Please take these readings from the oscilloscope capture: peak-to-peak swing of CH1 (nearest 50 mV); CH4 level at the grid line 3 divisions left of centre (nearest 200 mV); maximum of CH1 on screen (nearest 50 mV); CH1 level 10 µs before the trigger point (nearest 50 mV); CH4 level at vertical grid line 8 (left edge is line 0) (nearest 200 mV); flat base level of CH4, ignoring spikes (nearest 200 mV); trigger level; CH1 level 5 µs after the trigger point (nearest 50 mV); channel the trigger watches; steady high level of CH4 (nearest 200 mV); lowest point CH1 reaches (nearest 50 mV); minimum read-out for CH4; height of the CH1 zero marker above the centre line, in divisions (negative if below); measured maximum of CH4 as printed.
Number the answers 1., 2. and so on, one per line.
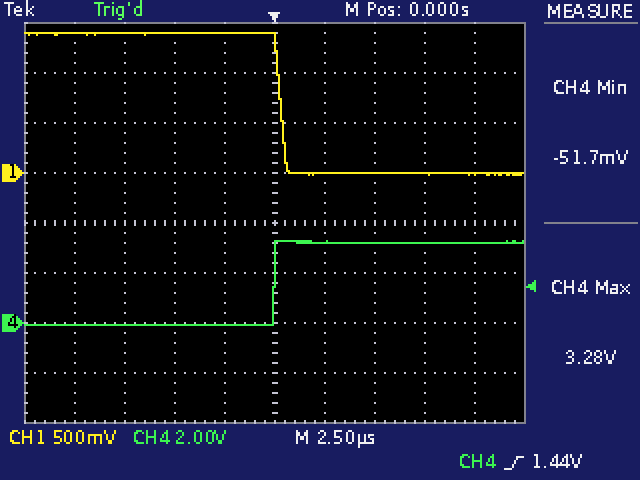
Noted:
1. 1.40 V
2. 0.0 V
3. 1.40 V
4. 1.40 V
5. 3.2 V
6. 0.0 V
7. 1.44 V
8. 0 mV
9. CH4
10. 3.2 V
11. 0 mV
12. -51.7 mV
13. +1.0 div
14. 3.28 V
